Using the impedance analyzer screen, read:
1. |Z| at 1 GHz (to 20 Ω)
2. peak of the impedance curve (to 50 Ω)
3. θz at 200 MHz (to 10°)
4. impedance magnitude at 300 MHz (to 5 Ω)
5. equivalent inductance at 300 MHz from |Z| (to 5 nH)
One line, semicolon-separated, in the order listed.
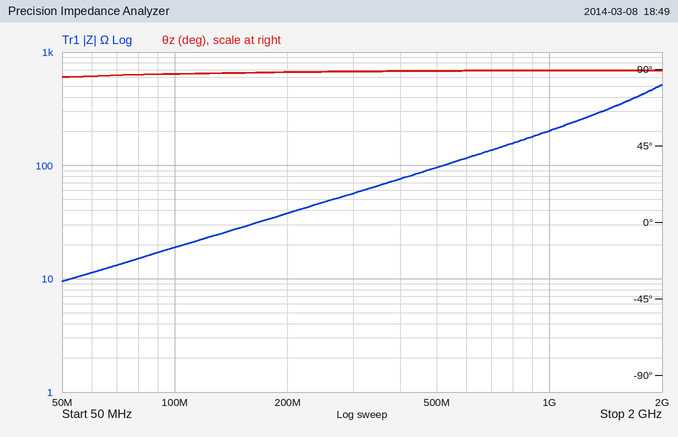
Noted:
200 Ω; 500 Ω; 90°; 55 Ω; 30 nH
